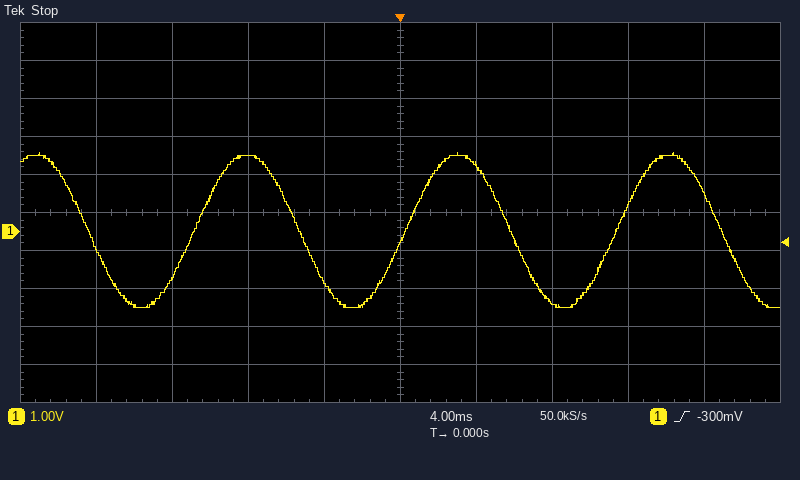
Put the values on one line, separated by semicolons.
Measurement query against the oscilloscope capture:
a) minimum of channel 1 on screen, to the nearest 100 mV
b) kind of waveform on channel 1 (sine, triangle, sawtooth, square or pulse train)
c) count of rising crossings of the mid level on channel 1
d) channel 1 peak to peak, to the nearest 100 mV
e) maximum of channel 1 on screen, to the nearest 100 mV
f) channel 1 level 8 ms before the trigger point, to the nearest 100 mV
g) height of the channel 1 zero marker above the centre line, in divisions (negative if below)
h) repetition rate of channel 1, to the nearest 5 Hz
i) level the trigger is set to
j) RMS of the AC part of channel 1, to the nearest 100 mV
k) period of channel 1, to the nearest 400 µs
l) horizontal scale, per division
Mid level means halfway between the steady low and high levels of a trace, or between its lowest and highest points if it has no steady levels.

-2.0 V; sine; 3; 4.1 V; 2.1 V; 2.0 V; -0.5 div; 90 Hz; -300 mV; 1.4 V; 11.2 ms; 4 ms
